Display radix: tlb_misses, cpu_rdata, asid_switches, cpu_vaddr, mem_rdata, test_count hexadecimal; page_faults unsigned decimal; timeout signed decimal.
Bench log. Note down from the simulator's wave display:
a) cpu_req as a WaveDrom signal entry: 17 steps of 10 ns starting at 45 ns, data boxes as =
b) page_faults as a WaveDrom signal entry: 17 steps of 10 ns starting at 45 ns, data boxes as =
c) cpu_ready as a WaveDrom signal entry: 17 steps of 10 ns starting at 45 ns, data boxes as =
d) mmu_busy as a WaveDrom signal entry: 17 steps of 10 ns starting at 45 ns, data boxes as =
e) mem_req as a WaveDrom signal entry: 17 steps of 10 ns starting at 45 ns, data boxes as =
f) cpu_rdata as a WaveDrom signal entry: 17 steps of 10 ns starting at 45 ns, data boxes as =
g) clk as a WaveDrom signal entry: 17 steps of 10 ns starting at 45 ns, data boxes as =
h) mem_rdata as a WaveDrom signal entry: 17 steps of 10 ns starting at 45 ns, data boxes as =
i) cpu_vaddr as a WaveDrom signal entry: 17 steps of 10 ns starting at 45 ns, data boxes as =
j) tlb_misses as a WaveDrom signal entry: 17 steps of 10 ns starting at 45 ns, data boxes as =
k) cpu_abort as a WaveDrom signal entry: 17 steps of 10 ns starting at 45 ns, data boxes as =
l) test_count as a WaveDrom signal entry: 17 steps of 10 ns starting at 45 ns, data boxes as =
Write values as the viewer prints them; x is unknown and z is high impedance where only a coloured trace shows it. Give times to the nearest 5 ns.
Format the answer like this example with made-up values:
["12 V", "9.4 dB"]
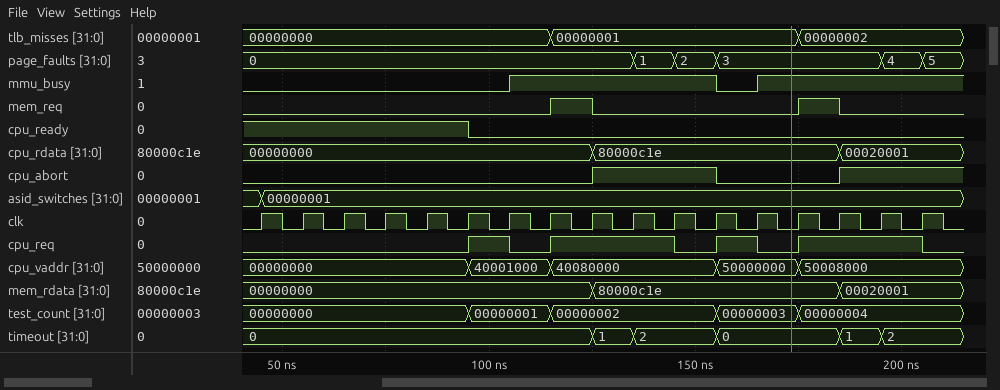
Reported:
["{name: 'cpu_req', wave: '0....101..0101..0'}", "{name: 'page_faults', wave: '=........===...==', data: '0 1 2 3 4 5'}", "{name: 'cpu_ready', wave: '1....0...........'}", "{name: 'mmu_busy', wave: '0.....1....01....'}", "{name: 'mem_req', wave: '0......10....10..'}", "{name: 'cpu_rdata', wave: '=.......=.....=..', data: '00000000 80000c1e 00020001'}", "{name: 'clk', wave: 'p................'}", "{name: 'mem_rdata', wave: '=.......=.....=..', data: '00000000 80000c1e 00020001'}", "{name: 'cpu_vaddr', wave: '=....=.=...=.=...', data: '00000000 40001000 40080000 50000000 50008000'}", "{name: 'tlb_misses', wave: '=......=.....=...', data: '00000000 00000001 00000002'}", "{name: 'cpu_abort', wave: '0.......1..0..1..'}", "{name: 'test_count', wave: '=....=.=...=.=...', data: '00000000 00000001 00000002 00000003 00000004'}"]
